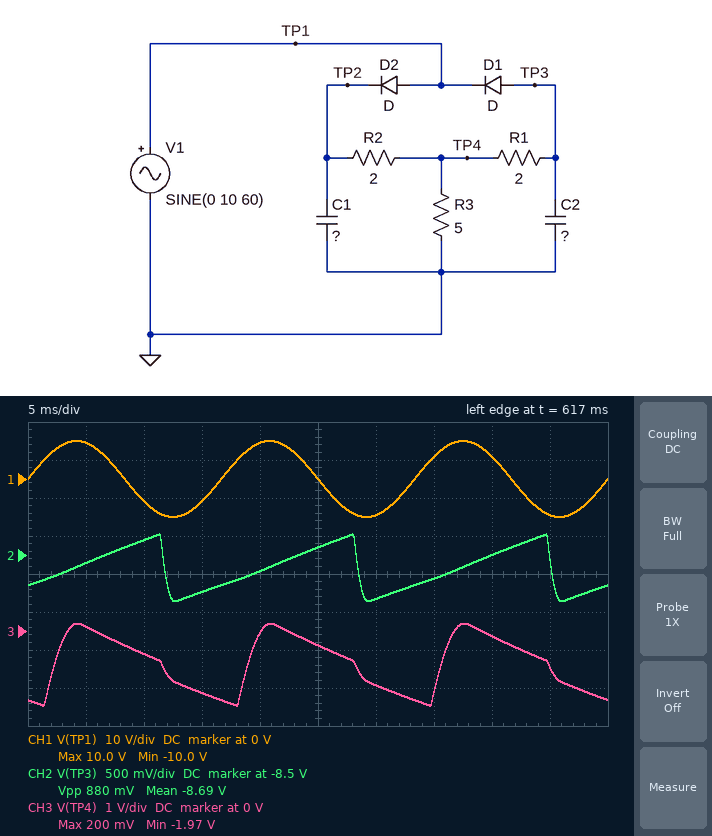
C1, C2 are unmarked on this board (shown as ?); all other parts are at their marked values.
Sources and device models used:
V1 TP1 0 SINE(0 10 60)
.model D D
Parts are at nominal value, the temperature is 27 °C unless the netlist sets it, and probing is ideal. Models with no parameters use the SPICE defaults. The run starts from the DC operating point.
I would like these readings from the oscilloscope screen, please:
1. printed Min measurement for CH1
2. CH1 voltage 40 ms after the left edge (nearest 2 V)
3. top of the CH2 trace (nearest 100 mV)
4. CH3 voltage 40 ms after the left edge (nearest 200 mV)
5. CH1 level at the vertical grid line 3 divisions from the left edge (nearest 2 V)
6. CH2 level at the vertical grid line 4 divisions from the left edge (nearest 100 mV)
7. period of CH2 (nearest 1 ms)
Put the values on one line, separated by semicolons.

-10.0 V; 6 V; -8.2 V; -200 mV; -6 V; -8.7 V; 17 ms
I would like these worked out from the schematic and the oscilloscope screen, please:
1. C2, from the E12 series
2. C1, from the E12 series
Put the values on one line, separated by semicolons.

68 mF; 10 mF
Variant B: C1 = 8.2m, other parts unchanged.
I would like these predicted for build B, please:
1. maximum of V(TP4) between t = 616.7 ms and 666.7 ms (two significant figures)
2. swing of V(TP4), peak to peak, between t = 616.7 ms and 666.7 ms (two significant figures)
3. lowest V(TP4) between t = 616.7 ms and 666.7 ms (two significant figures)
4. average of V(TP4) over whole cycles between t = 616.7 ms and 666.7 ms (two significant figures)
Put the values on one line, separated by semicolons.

190 mV; 2.5 V; -2.3 V; -1.0 V
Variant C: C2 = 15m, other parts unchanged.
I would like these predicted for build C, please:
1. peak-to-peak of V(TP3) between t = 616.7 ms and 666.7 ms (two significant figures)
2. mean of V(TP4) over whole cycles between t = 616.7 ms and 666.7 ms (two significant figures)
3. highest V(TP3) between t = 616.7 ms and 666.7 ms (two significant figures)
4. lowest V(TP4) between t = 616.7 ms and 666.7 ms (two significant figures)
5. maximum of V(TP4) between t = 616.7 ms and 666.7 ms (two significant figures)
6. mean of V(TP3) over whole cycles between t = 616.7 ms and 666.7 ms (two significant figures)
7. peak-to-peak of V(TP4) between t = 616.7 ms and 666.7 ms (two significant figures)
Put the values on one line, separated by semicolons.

3.4 V; -290 mV; -5.7 V; -1.5 V; 830 mV; -7.5 V; 2.3 V
